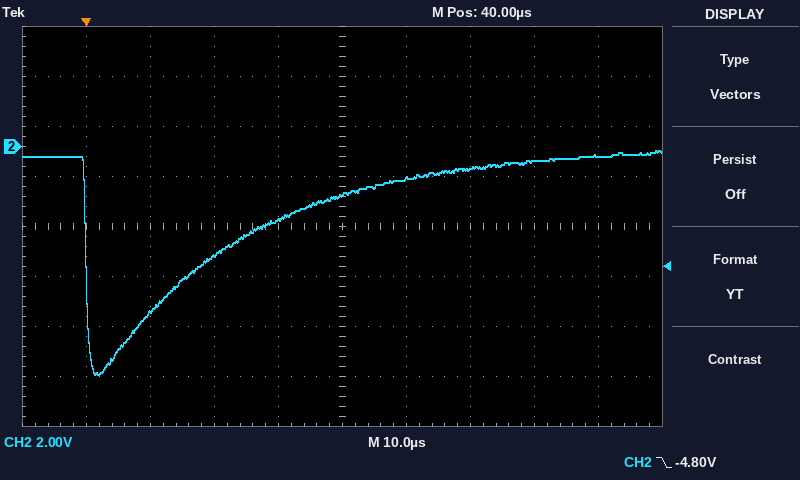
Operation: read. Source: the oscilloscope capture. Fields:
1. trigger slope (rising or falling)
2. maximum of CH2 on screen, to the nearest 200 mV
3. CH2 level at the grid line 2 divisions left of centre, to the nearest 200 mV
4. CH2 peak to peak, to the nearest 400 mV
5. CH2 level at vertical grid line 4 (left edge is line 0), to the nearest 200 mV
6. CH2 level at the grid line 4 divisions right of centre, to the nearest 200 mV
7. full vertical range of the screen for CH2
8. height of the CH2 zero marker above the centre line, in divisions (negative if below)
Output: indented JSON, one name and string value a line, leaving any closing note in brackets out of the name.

{
  "trigger slope": "falling",
  "maximum of CH2 on screen, to the nearest 200 mV": "-200 mV",
  "CH2 level at the grid line 2 divisions left of centre, to the nearest 200 mV": "-4.4 V",
  "CH2 peak to peak, to the nearest 400 mV": "8.8 V",
  "CH2 level at vertical grid line 4 (left edge is line 0), to the nearest 200 mV": "-3.0 V",
  "CH2 level at the grid line 4 divisions right of centre, to the nearest 200 mV": "-400 mV",
  "full vertical range of the screen for CH2": "16 V",
  "height of the CH2 zero marker above the centre line, in divisions": "+1.6 div"
}
